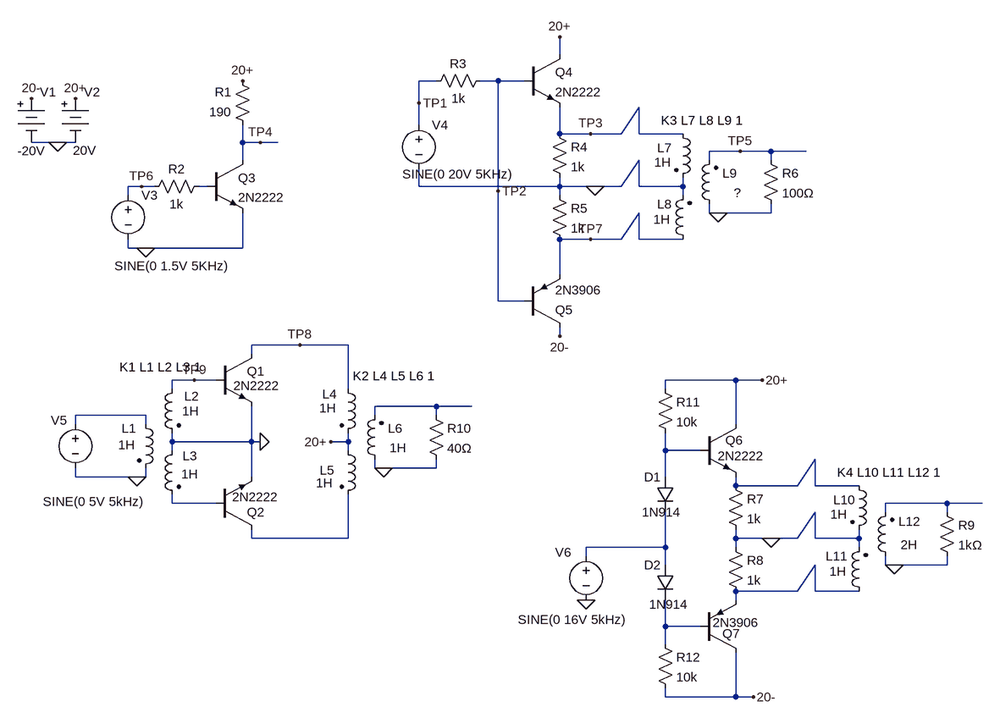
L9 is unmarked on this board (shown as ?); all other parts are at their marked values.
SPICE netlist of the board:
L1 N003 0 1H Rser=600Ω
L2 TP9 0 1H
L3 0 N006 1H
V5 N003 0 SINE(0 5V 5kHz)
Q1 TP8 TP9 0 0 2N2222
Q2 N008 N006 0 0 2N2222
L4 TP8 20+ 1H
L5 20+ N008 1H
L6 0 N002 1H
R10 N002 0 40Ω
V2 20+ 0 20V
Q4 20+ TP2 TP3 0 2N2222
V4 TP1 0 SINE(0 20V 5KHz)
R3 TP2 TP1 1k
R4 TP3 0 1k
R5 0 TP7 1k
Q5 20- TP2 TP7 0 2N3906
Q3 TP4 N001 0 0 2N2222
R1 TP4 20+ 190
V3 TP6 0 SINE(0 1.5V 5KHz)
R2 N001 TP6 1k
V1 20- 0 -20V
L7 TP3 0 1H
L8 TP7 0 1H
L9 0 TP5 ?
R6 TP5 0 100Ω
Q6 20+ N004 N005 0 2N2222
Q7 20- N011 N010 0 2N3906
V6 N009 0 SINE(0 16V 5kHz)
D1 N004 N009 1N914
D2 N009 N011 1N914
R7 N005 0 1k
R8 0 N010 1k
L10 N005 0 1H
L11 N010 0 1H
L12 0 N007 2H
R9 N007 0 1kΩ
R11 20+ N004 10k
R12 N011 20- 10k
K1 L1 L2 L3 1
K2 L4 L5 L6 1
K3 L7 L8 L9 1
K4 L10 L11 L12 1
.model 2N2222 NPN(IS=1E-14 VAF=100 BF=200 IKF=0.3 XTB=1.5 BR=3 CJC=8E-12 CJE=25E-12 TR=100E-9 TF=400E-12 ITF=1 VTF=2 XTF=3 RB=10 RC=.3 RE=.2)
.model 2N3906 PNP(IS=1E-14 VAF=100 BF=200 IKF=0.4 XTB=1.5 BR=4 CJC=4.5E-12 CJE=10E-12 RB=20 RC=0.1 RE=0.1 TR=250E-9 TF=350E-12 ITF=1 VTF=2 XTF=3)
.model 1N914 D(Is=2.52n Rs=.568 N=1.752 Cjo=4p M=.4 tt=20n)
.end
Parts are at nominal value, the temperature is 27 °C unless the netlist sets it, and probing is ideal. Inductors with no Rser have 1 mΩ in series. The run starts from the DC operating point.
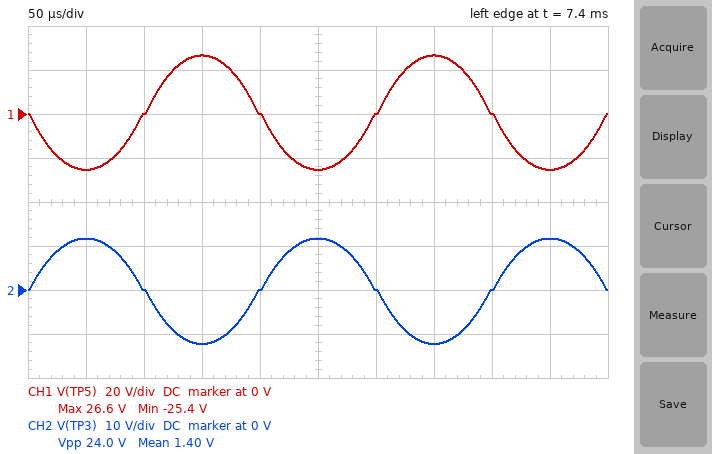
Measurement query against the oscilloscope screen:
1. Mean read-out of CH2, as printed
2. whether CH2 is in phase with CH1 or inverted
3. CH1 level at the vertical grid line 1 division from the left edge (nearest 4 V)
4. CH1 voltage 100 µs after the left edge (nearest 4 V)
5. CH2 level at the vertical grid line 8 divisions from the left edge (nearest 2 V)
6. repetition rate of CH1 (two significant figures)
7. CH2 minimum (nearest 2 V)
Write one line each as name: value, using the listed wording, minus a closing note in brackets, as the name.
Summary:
Mean read-out of CH2, as printed: 1.40 V
whether CH2 is in phase with CH1 or inverted: inverted
CH1 level at the vertical grid line 1 division from the left edge: -24 V
CH1 voltage 100 µs after the left edge: 0 V
CH2 level at the vertical grid line 8 divisions from the left edge: 0 V
repetition rate of CH1: 5.0 kHz
CH2 minimum: -12 V
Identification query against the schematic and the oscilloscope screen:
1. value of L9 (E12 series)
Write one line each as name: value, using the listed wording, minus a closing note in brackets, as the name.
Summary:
value of L9: 4.7 H
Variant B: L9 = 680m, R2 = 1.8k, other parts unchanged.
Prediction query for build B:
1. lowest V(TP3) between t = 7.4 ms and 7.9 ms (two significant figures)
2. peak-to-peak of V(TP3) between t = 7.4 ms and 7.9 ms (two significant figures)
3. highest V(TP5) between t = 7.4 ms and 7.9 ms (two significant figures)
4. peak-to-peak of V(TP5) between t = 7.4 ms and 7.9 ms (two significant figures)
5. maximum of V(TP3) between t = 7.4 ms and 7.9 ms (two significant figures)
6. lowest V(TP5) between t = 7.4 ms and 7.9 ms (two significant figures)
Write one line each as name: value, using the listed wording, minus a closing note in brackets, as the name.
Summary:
lowest V(TP3) between t = 7.4 ms and 7.9 ms: -18 V
peak-to-peak of V(TP3) between t = 7.4 ms and 7.9 ms: 36 V
highest V(TP5) between t = 7.4 ms and 7.9 ms: 15 V
peak-to-peak of V(TP5) between t = 7.4 ms and 7.9 ms: 30 V
maximum of V(TP3) between t = 7.4 ms and 7.9 ms: 18 V
lowest V(TP5) between t = 7.4 ms and 7.9 ms: -15 V
